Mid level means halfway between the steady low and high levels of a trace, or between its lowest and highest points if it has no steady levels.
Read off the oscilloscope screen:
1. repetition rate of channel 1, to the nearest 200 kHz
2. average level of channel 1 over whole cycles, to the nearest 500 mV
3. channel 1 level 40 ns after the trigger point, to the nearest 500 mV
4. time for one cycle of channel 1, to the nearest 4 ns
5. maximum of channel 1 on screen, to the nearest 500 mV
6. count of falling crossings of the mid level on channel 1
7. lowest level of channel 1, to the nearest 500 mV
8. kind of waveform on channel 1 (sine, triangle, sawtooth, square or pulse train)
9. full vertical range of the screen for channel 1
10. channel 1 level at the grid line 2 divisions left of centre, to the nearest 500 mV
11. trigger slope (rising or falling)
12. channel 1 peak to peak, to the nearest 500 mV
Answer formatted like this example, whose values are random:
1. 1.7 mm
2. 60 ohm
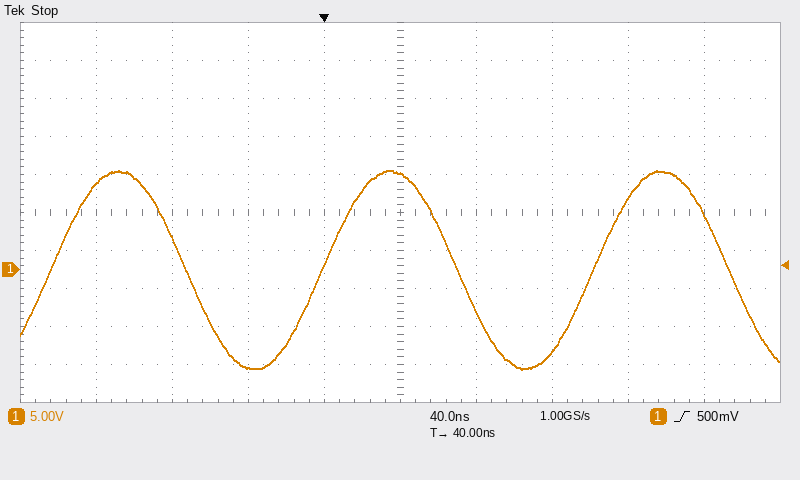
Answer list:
1. 7.0 MHz
2. 0.0 V
3. 12.5 V
4. 144 ns
5. 13.0 V
6. 3
7. -13.0 V
8. sine
9. 50 V
10. -13.0 V
11. rising
12. 26.0 V
